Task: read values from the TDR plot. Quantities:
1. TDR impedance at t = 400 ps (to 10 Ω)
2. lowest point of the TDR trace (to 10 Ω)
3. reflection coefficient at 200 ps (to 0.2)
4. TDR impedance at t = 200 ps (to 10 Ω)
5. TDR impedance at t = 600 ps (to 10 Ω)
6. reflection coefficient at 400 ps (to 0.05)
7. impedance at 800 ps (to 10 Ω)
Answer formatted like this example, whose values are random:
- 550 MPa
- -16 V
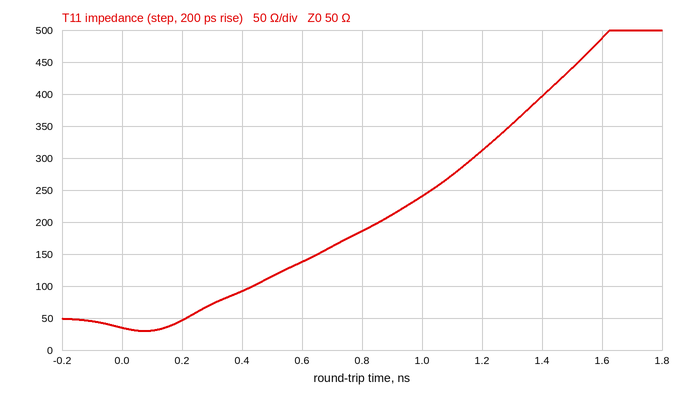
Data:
- 90 Ω
- 30 Ω
- 0.0
- 50 Ω
- 140 Ω
- +0.30
- 190 Ω
